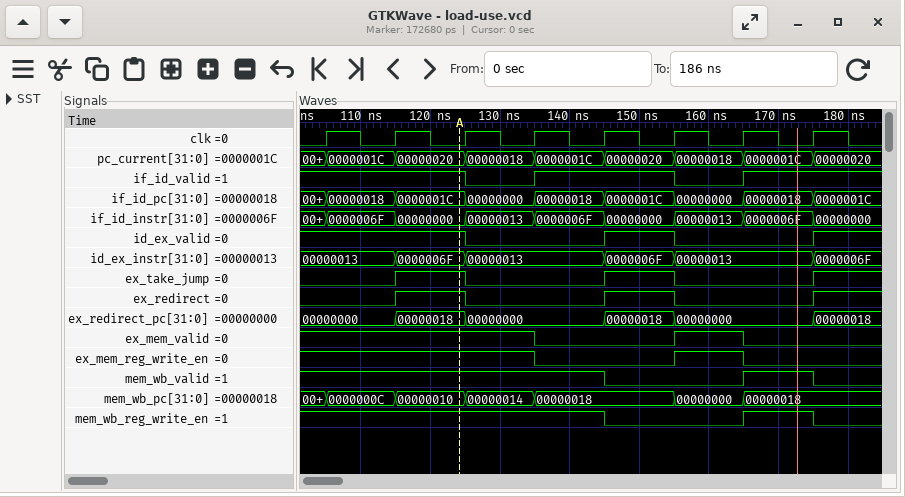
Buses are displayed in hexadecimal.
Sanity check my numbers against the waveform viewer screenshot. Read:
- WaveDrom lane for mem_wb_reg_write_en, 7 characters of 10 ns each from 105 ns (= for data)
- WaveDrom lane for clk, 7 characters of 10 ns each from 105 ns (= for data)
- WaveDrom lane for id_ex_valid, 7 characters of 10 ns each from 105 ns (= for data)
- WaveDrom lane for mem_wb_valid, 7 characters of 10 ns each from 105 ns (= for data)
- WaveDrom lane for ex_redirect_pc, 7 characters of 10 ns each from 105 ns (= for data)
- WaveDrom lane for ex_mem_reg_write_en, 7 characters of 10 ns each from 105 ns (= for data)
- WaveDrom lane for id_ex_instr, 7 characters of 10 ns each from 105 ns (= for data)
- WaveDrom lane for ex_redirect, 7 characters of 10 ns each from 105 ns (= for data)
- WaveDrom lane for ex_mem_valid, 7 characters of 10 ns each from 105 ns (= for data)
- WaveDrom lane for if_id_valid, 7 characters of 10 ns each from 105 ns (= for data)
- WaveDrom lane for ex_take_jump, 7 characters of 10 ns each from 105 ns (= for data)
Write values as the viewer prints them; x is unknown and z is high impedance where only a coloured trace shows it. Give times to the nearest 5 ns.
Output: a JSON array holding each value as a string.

["{name: 'mem_wb_reg_write_en', wave: '1...0.1'}", "{name: 'clk', wave: 'p......'}", "{name: 'id_ex_valid', wave: '1.0.10.'}", "{name: 'mem_wb_valid', wave: '1...0.1'}", "{name: 'ex_redirect_pc', wave: '===.==.', data: '00000000 00000018 00000000 00000018 00000000'}", "{name: 'ex_mem_reg_write_en', wave: '1..0.10'}", "{name: 'id_ex_instr', wave: '===.==.', data: '00000013 0000006F 00000013 0000006F 00000013'}", "{name: 'ex_redirect', wave: '010.10.'}", "{name: 'ex_mem_valid', wave: '1..0.10'}", "{name: 'if_id_valid', wave: '1.01.01'}", "{name: 'ex_take_jump', wave: '010.10.'}"]
